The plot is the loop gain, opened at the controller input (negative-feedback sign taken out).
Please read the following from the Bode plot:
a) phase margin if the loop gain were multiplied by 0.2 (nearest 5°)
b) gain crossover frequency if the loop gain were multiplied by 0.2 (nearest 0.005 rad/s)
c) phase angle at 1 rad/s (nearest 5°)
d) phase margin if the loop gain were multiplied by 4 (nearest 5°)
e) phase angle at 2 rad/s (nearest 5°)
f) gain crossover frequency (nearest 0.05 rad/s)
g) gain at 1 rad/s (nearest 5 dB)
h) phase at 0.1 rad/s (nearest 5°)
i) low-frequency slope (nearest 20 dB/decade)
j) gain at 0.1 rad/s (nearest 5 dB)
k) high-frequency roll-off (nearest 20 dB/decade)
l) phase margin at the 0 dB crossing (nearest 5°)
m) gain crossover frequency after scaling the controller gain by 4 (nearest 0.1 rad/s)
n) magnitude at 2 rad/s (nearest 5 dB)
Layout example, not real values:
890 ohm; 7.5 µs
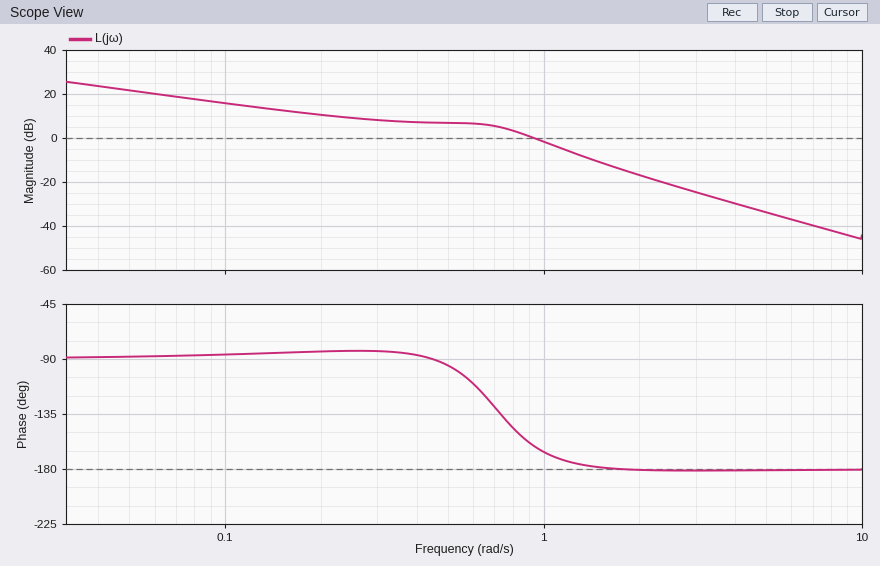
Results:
95°; 0.125 rad/s; -165°; 0°; -180°; 0.95 rad/s; 0 dB; -85°; -20 dB/decade; 15 dB; -40 dB/decade; 20°; 1.6 rad/s; -15 dB
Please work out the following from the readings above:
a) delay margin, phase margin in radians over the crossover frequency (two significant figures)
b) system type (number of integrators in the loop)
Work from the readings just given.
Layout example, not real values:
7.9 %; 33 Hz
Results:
0.37 s; 1
